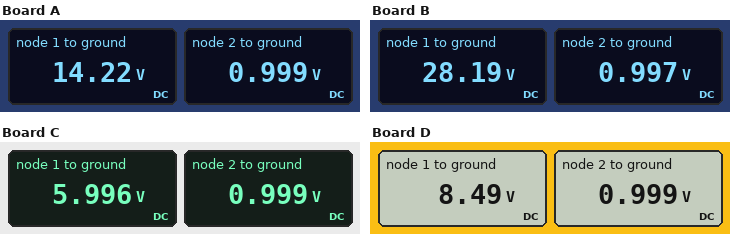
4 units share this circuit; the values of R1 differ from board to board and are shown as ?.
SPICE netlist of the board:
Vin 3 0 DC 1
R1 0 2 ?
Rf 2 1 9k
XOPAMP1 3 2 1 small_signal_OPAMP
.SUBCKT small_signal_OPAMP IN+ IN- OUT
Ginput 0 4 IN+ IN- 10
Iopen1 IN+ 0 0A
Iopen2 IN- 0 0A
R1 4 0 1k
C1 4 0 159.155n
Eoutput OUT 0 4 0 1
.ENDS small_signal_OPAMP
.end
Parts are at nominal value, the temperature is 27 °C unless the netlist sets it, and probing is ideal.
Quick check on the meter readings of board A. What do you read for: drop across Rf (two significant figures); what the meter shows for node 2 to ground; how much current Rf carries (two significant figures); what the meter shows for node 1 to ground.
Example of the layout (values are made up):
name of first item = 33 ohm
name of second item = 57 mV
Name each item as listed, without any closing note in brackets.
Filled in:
drop across Rf = 13 V
what the meter shows for node 2 to ground = 0.999 V
how much current Rf carries = 1.5 mA
what the meter shows for node 1 to ground = 14.22 V
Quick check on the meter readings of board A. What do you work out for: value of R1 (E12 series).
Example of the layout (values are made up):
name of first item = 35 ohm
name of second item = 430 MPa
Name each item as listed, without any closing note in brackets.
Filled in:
value of R1 = 680 Ω
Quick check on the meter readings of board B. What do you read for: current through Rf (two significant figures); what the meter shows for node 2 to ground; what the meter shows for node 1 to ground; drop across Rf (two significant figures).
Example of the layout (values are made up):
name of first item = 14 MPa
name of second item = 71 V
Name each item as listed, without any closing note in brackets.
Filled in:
current through Rf = 3.0 mA
what the meter shows for node 2 to ground = 0.997 V
what the meter shows for node 1 to ground = 28.19 V
drop across Rf = 27 V
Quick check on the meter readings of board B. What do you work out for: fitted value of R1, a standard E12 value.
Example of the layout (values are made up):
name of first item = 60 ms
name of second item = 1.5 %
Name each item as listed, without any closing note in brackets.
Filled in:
fitted value of R1, a standard E12 value = 330 Ω
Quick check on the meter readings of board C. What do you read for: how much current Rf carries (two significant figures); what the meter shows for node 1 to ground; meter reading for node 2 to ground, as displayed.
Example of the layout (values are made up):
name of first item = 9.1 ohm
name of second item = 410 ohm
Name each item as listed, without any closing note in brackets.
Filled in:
how much current Rf carries = 560 µA
what the meter shows for node 1 to ground = 5.996 V
meter reading for node 2 to ground, as displayed = 0.999 V
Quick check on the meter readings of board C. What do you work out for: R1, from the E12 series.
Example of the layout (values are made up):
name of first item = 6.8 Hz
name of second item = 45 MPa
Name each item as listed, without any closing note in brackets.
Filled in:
R1, from the E12 series = 1.8 kΩ
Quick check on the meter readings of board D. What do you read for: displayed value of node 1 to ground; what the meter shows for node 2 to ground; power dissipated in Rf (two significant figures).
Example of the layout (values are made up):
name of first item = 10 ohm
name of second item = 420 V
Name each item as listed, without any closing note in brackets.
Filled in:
displayed value of node 1 to ground = 8.49 V
what the meter shows for node 2 to ground = 0.999 V
power dissipated in Rf = 6.2 mW
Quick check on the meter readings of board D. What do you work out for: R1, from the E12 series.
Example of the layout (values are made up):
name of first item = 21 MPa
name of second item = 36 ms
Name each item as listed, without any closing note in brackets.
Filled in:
R1, from the E12 series = 1.2 kΩ
